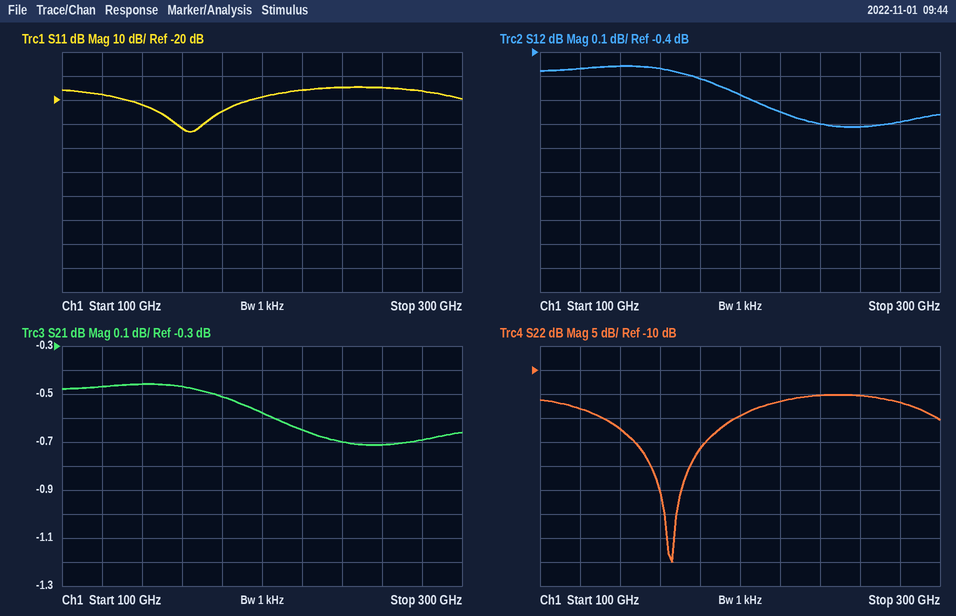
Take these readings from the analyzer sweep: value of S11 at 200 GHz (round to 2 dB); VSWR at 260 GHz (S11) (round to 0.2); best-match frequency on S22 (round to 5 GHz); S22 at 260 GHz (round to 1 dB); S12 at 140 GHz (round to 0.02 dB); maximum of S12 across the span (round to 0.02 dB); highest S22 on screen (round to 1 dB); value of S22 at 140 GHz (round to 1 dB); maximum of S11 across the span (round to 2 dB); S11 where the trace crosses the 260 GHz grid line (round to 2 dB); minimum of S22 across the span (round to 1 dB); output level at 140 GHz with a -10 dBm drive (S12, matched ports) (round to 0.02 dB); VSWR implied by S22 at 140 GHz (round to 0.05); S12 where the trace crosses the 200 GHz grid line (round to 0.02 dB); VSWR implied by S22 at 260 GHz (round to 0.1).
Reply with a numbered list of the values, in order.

1. -18 dB
2. 1.4
3. 165 GHz
4. -15 dB
5. -0.46 dB
6. -0.46 dB
7. -15 dB
8. -22 dB
9. -14 dB
10. -14 dB
11. -50 dB
12. -10.46 dBm
13. 1.15
14. -0.58 dB
15. 1.4
